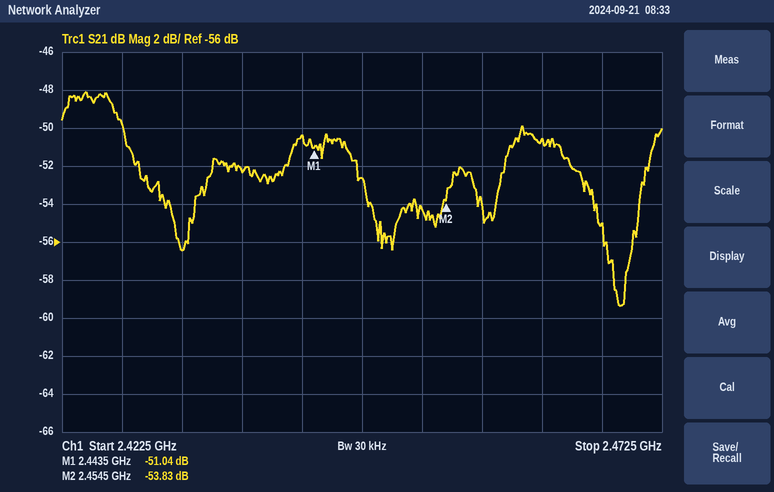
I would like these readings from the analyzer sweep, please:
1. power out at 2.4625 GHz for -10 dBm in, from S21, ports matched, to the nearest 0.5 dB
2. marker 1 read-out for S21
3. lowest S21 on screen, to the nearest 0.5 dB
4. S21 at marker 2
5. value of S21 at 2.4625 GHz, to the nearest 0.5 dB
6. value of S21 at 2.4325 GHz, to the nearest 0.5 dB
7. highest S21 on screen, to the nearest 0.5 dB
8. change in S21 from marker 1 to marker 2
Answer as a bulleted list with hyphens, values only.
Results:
- -60.5 dBm
- -51.04 dB
- -59.5 dB
- -53.83 dB
- -50.5 dB
- -56.5 dB
- -48.0 dB
- -2.79 dB
